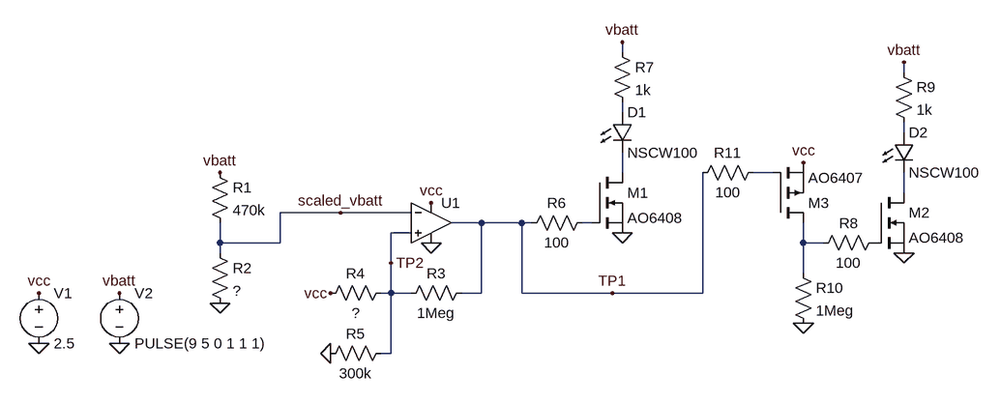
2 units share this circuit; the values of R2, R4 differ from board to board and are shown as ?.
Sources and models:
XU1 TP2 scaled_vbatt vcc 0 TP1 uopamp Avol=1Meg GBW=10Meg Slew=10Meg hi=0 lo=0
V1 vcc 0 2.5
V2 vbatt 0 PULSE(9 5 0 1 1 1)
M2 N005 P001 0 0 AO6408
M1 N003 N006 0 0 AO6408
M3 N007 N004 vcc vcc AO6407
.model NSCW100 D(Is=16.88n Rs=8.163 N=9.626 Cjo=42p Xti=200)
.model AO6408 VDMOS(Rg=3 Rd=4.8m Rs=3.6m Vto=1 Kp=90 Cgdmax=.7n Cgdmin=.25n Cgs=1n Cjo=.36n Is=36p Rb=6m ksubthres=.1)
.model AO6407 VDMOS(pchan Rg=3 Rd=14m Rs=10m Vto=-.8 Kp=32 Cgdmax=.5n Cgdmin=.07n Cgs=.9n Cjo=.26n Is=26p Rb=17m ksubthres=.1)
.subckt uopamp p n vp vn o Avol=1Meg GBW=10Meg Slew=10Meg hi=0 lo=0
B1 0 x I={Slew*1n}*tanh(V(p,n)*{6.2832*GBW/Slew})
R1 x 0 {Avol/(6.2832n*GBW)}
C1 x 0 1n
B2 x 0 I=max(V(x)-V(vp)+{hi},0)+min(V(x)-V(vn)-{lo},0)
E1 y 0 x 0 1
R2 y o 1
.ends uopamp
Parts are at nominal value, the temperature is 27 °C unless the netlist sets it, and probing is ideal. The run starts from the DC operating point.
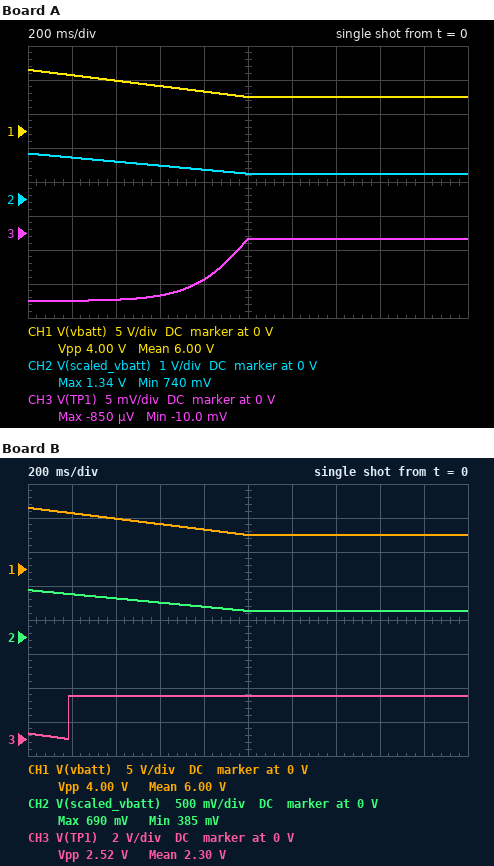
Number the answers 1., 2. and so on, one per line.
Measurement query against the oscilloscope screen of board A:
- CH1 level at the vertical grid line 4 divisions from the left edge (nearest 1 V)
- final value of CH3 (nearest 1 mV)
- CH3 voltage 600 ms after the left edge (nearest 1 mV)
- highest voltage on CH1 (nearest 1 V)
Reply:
1. 6 V
2. -1 mV
3. -9 mV
4. 9 V
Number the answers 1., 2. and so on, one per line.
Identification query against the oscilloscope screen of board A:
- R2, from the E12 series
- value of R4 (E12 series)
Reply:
1. 82 kΩ
2. 560 kΩ
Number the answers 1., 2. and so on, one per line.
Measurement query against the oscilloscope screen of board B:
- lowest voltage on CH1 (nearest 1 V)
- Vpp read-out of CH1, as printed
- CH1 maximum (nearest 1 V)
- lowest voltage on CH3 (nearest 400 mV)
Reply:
1. 5 V
2. 4.00 V
3. 9 V
4. 0 V
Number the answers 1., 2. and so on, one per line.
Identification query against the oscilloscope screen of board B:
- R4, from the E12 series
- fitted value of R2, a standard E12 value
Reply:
1. 680 kΩ
2. 39 kΩ
